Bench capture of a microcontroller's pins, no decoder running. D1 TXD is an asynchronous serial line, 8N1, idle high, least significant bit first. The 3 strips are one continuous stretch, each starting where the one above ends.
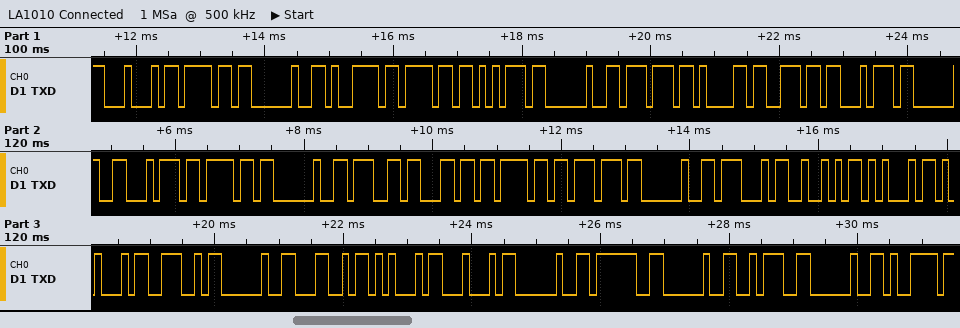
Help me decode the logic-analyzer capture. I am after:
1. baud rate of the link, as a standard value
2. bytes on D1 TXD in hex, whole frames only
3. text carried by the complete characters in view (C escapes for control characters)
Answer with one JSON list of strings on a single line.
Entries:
["9600 baud", "44 6F 20 79 6F 75 20 77 61 6E 74 20 74 6F 20 67 6C 6F 77 20 47 52 45 45 4E 20 4C 45 44 20 3F 20 3A 20 79", "\"Do you want to glow GREEN LED ? : y\""]
